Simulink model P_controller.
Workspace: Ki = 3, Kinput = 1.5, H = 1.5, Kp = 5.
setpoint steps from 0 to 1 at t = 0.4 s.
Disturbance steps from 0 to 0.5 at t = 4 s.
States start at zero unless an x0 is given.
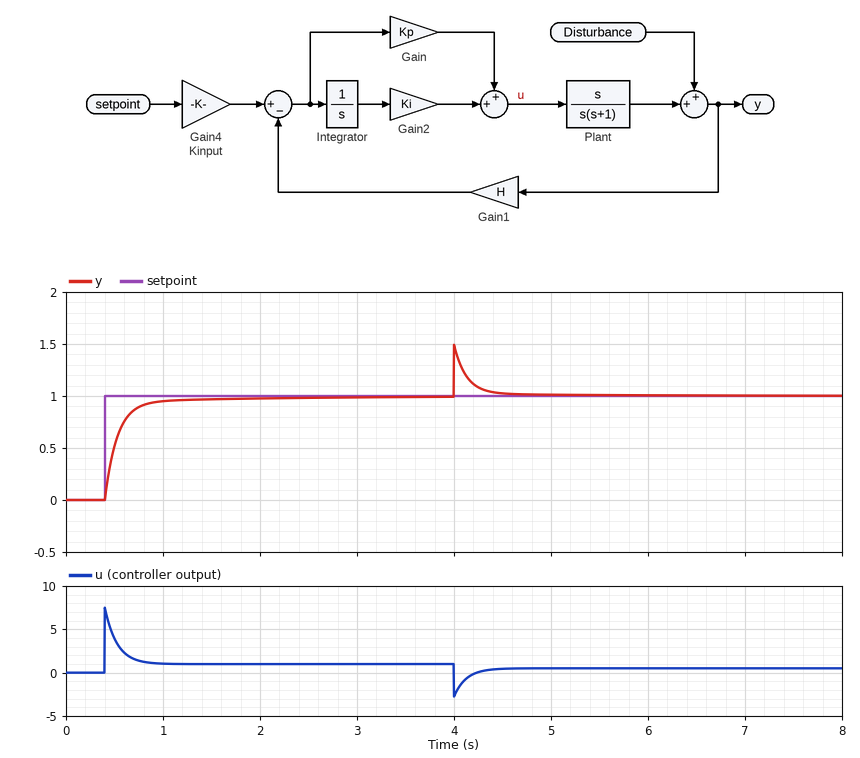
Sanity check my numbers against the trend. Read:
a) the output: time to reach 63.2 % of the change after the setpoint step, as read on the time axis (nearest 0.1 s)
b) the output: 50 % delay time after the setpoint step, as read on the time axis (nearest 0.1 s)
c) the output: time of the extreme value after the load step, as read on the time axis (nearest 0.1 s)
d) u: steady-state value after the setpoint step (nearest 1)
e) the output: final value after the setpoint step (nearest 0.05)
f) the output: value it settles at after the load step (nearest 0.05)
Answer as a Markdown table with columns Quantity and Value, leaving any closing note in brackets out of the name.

| Quantity | Value |
|---|---|
| the output: time to reach 63.2 % of the change after the setpoint step, as read on the time axis | 0.5 s |
| the output: 50 % delay time after the setpoint step, as read on the time axis | 0.5 s |
| the output: time of the extreme value after the load step, as read on the time axis | 4.0 s |
| u: steady-state value after the setpoint step | 1 |
| the output: final value after the setpoint step | 1.00 |
| the output: value it settles at after the load step | 1.00 |
